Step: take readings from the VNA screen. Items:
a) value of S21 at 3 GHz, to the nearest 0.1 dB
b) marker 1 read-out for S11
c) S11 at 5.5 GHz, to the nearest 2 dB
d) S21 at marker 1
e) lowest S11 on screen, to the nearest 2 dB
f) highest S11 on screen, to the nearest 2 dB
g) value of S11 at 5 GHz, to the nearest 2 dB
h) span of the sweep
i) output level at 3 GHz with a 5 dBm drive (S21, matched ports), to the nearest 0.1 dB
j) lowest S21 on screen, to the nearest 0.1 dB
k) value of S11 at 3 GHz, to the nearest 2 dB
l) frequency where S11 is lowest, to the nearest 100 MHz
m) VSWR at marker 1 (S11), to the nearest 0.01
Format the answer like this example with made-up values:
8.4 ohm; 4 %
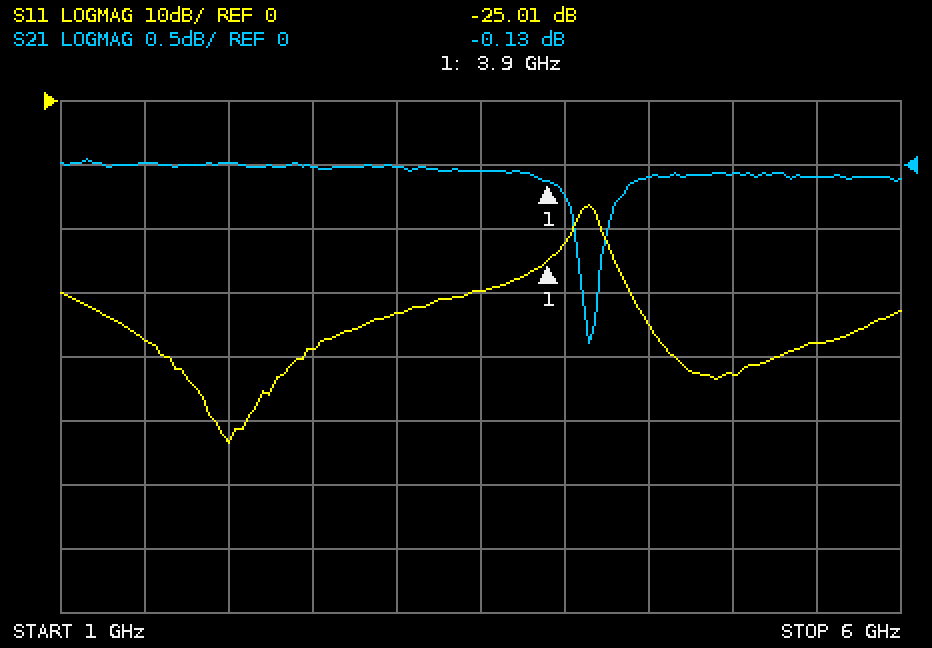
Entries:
0.0 dB; -25.01 dB; -38 dB; -0.13 dB; -54 dB; -16 dB; -42 dB; 5 GHz; 5.0 dBm; -1.4 dB; -34 dB; 2.0 GHz; 1.12
